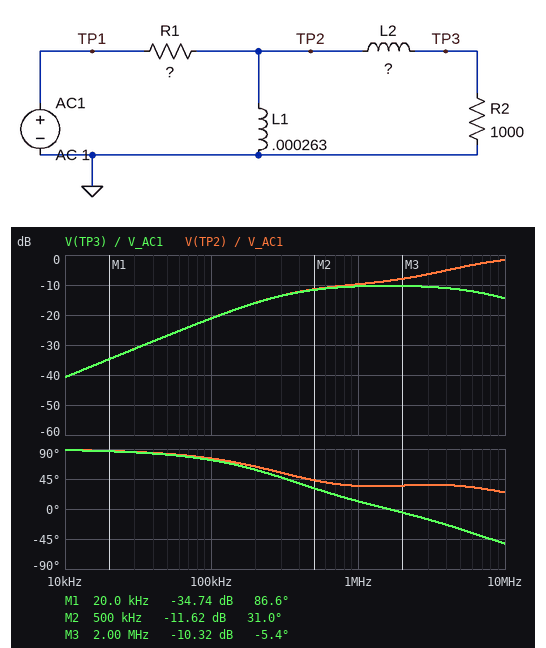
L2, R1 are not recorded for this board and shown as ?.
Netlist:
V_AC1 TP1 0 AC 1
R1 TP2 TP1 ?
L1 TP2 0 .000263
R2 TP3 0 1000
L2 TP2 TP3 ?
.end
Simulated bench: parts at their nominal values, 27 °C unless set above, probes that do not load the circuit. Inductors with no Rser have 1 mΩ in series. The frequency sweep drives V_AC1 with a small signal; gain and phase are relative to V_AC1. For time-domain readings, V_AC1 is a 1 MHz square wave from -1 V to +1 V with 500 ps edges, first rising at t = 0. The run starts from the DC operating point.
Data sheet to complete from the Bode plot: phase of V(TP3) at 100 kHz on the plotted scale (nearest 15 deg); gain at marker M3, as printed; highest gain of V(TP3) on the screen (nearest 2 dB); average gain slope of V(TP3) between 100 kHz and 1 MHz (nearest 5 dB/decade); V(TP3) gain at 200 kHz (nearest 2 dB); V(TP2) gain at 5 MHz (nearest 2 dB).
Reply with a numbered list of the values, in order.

1. 75 deg
2. -10.32 dB
3. -10 dB
4. 10 dB/decade
5. -16 dB
6. -4 dB
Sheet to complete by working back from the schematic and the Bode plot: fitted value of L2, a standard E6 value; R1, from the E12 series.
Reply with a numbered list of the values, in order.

1. 68 µH
2. 1.8 kΩ
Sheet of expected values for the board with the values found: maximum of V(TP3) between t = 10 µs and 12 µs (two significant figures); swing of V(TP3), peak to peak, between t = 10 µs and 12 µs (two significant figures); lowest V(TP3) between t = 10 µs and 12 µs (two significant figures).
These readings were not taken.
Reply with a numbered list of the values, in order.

1. 410 mV
2. 810 mV
3. -410 mV
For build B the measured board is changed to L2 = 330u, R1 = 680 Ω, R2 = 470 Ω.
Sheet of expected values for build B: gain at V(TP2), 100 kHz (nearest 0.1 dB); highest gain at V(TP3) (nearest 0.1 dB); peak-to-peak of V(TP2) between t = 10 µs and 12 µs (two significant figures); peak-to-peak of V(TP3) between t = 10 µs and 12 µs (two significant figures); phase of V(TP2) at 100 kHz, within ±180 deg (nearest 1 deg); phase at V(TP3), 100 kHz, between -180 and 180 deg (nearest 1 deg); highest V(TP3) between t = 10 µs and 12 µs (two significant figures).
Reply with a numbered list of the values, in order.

1. -14.2 dB
2. -12.6 dB
3. 3.5 V
4. 430 mV
5. 65 deg
6. 41 deg
7. 210 mV
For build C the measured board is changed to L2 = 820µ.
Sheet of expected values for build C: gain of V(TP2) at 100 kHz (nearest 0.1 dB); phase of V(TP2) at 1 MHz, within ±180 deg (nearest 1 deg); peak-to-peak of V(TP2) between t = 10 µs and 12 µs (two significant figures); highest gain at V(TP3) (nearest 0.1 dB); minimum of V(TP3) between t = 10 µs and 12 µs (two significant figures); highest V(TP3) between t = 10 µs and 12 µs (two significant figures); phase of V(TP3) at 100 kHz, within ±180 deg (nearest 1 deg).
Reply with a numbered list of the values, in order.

1. -21.5 dB
2. 53 deg
3. 3.9 V
4. -18.5 dB
5. -120 mV
6. 120 mV
7. 51 deg
